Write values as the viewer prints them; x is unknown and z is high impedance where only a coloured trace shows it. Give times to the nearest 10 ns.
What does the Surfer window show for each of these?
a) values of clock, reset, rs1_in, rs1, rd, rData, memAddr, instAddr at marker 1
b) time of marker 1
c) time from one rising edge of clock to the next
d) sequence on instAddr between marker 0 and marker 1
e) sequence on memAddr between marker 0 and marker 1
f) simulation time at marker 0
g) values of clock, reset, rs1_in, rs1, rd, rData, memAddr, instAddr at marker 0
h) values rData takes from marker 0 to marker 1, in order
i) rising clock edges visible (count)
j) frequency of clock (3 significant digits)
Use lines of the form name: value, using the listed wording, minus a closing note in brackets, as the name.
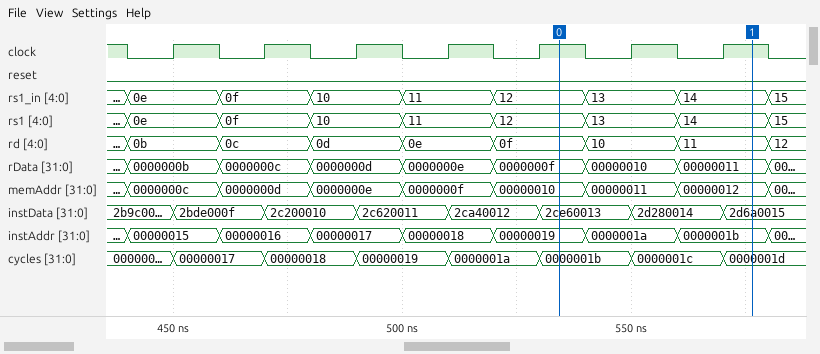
values of clock, reset, rs1_in, rs1, rd, rData, memAddr, instAddr at marker 1: clock=1, reset=0, rs1_in=14, rs1=14, rd=11, rData=00000011, memAddr=00000012, instAddr=0000001b
time of marker 1: 580 ns
time from one rising edge of clock to the next: 20 ns
sequence on instAddr between marker 0 and marker 1: 00000019, 0000001a, 0000001b
sequence on memAddr between marker 0 and marker 1: 00000010, 00000011, 00000012
simulation time at marker 0: 530 ns
values of clock, reset, rs1_in, rs1, rd, rData, memAddr, instAddr at marker 0: clock=1, reset=0, rs1_in=12, rs1=12, rd=0f, rData=0000000f, memAddr=00000010, instAddr=00000019
values rData takes from marker 0 to marker 1, in order: 0000000f, 00000010, 00000011
rising clock edges visible: 7
frequency of clock: 50.0 MHz
